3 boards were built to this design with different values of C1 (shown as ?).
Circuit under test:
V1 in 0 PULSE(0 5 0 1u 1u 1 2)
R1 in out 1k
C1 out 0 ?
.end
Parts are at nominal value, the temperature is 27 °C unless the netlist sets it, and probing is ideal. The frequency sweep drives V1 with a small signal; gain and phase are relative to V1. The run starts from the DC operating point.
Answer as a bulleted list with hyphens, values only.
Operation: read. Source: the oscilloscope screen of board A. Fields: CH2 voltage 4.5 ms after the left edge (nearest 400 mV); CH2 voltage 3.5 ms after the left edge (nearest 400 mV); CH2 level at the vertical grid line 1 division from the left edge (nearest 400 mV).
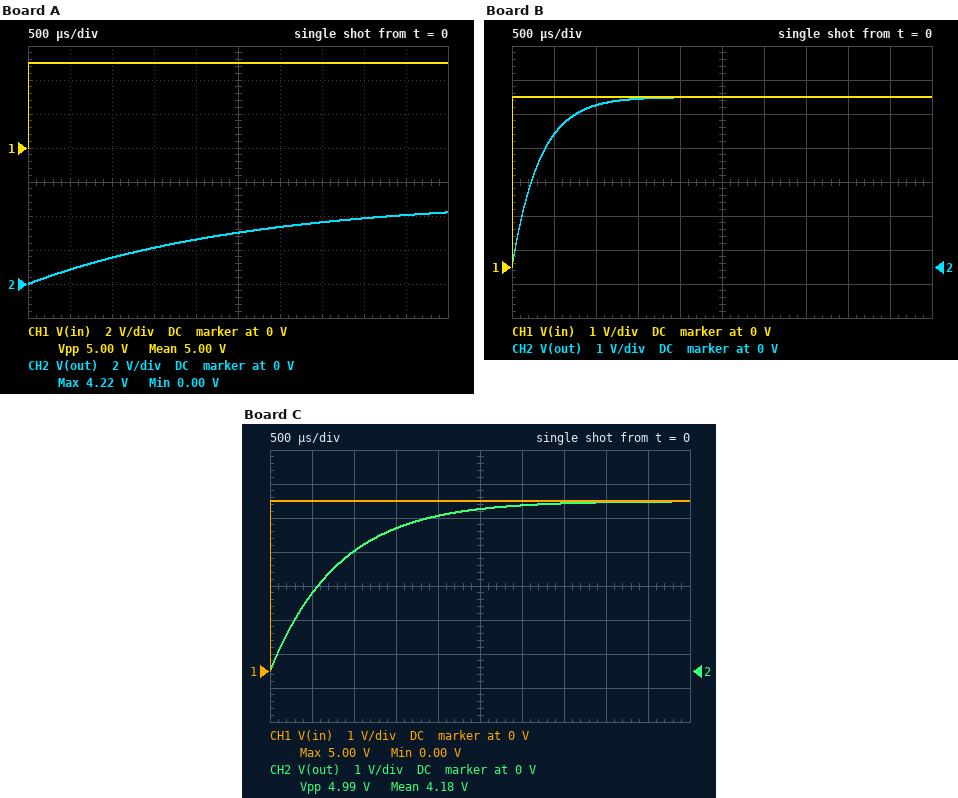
- 4.0 V
- 3.6 V
- 800 mV
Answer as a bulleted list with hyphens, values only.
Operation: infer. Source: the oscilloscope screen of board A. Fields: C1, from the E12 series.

- 2.7 µF
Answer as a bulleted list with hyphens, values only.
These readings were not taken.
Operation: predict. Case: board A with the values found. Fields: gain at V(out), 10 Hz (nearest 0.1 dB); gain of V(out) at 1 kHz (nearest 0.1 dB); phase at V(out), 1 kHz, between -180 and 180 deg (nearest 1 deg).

- -0.1 dB
- -24.6 dB
- -87 deg
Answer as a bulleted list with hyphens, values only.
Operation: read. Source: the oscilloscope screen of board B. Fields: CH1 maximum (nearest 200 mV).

- 5.0 V
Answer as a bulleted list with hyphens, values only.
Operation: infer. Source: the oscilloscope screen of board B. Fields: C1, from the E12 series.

- 330 nF
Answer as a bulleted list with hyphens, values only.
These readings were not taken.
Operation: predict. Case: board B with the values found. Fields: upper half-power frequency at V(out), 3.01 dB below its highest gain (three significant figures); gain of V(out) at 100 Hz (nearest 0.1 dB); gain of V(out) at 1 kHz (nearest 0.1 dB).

- 482 Hz
- -0.2 dB
- -7.2 dB
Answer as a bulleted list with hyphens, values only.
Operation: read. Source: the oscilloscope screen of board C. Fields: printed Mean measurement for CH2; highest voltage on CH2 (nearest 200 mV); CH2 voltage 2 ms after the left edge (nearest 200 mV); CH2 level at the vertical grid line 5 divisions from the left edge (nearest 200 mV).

- 4.18 V
- 5.0 V
- 4.6 V
- 4.8 V
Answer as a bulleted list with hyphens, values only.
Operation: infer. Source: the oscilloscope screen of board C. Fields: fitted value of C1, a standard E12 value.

- 820 nF
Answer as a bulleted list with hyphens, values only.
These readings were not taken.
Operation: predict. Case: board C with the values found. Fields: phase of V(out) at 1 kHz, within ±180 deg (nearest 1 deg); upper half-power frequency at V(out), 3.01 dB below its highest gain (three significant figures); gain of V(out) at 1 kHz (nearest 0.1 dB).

- -79 deg
- 194 Hz
- -14.4 dB
